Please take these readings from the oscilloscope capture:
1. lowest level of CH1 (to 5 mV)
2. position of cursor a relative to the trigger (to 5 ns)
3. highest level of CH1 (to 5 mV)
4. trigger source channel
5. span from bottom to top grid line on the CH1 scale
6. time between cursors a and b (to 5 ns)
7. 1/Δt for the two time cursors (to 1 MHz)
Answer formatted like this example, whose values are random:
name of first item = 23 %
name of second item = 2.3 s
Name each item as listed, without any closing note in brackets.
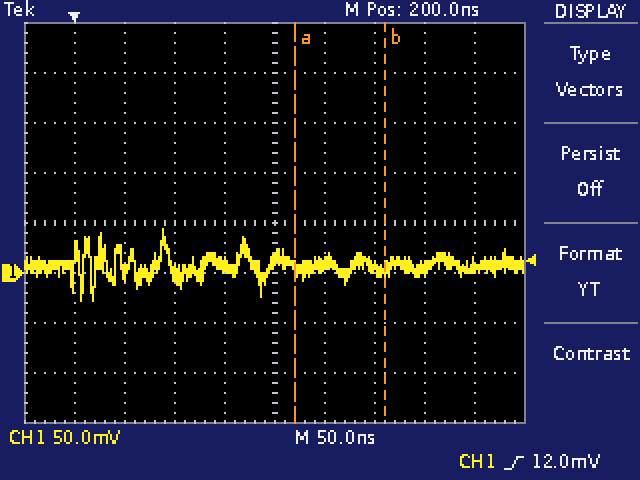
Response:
lowest level of CH1 = -30 mV
position of cursor a relative to the trigger = +220 ns
highest level of CH1 = 45 mV
trigger source channel = CH1
span from bottom to top grid line on the CH1 scale = 400 mV
time between cursors a and b = 90 ns
1/Δt for the two time cursors = 11 MHz
